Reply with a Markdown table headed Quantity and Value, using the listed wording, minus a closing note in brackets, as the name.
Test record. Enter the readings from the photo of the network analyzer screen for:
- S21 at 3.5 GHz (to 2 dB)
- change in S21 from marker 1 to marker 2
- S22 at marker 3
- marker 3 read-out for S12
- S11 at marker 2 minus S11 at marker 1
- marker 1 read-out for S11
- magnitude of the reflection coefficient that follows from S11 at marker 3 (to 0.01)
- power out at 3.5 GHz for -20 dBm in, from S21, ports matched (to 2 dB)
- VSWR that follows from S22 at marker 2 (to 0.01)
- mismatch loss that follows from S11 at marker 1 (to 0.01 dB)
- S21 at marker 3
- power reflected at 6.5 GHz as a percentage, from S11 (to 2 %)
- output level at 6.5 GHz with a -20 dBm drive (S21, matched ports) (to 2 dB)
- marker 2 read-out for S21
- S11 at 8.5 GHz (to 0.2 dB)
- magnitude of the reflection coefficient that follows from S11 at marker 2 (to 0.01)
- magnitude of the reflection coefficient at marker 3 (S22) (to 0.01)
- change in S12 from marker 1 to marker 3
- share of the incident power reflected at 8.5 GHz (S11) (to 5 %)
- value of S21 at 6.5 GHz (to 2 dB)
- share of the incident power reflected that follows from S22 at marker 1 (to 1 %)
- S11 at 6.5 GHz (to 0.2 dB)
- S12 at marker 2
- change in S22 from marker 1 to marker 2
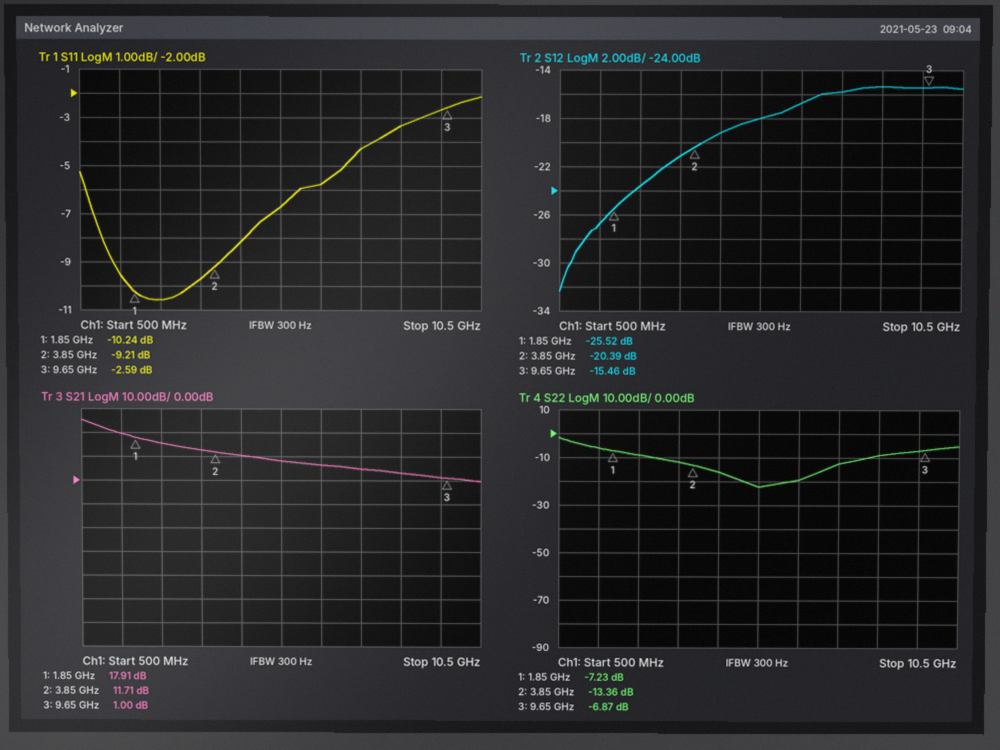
| Quantity | Value |
|---|---|
| S21 at 3.5 GHz | 12 dB |
| change in S21 from marker 1 to marker 2 | -6.20 dB |
| S22 at marker 3 | -6.87 dB |
| marker 3 read-out for S12 | -15.46 dB |
| S11 at marker 2 minus S11 at marker 1 | 1.03 dB |
| marker 1 read-out for S11 | -10.24 dB |
| magnitude of the reflection coefficient that follows from S11 at marker 3 | 0.74 |
| power out at 3.5 GHz for -20 dBm in, from S21, ports matched | -8 dBm |
| VSWR that follows from S22 at marker 2 | 1.55 |
| mismatch loss that follows from S11 at marker 1 | 0.43 dB |
| S21 at marker 3 | 1.00 dB |
| power reflected at 6.5 GHz as a percentage, from S11 | 26 % |
| output level at 6.5 GHz with a -20 dBm drive (S21, matched ports) | -14 dBm |
| marker 2 read-out for S21 | 11.71 dB |
| S11 at 8.5 GHz | -3.4 dB |
| magnitude of the reflection coefficient that follows from S11 at marker 2 | 0.35 |
| magnitude of the reflection coefficient at marker 3 (S22) | 0.45 |
| change in S12 from marker 1 to marker 3 | 10.06 dB |
| share of the incident power reflected at 8.5 GHz (S11) | 45 % |
| value of S21 at 6.5 GHz | 6 dB |
| share of the incident power reflected that follows from S22 at marker 1 | 19 % |
| S11 at 6.5 GHz | -5.8 dB |
| S12 at marker 2 | -20.39 dB |
| change in S22 from marker 1 to marker 2 | -6.13 dB |
